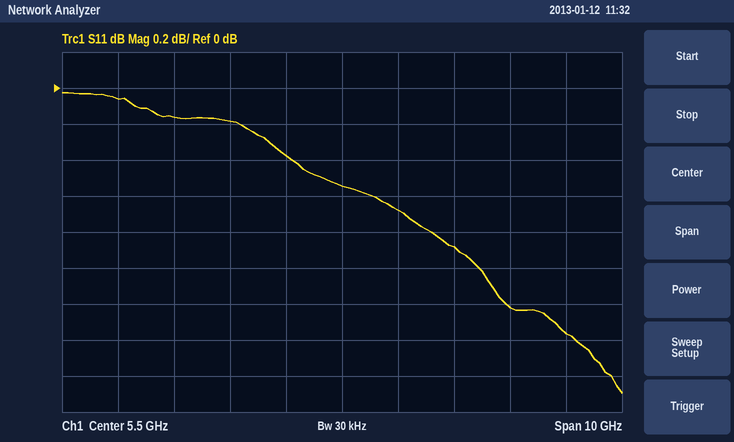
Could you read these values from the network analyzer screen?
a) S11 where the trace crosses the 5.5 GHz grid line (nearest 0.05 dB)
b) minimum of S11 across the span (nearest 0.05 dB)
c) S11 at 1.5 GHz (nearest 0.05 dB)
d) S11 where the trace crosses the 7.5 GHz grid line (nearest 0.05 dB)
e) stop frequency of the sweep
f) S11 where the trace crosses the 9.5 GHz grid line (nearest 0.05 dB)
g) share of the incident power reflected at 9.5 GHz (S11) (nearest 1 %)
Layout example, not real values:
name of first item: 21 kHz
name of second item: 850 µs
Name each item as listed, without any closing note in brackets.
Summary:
S11 where the trace crosses the 5.5 GHz grid line: -0.55 dB
minimum of S11 across the span: -1.70 dB
S11 at 1.5 GHz: -0.05 dB
S11 where the trace crosses the 7.5 GHz grid line: -0.90 dB
stop frequency of the sweep: 10.5 GHz
S11 where the trace crosses the 9.5 GHz grid line: -1.35 dB
share of the incident power reflected at 9.5 GHz (S11): 73 %
